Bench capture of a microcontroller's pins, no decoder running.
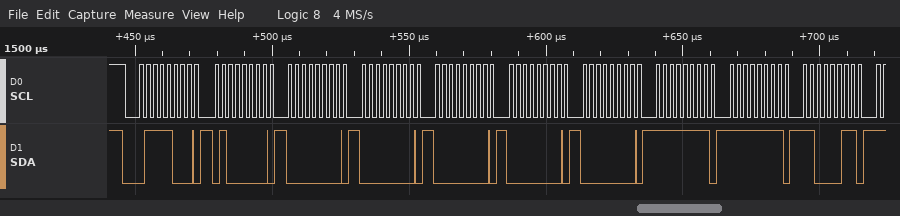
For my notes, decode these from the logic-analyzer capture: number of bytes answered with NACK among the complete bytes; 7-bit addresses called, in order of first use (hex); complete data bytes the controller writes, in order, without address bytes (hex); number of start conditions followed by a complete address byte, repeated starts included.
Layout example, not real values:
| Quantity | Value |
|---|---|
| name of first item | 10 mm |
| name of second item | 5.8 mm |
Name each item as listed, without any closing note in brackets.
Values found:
| Quantity | Value |
|---|---|
| number of bytes answered with NACK among the complete bytes | 0 |
| 7-bit addresses called, in order of first use | 0x3C |
| complete data bytes the controller writes, in order, without address bytes | 40 00 00 00 00 00 FF FF C3 |
| number of start conditions followed by a complete address byte, repeated starts included | 1 |
